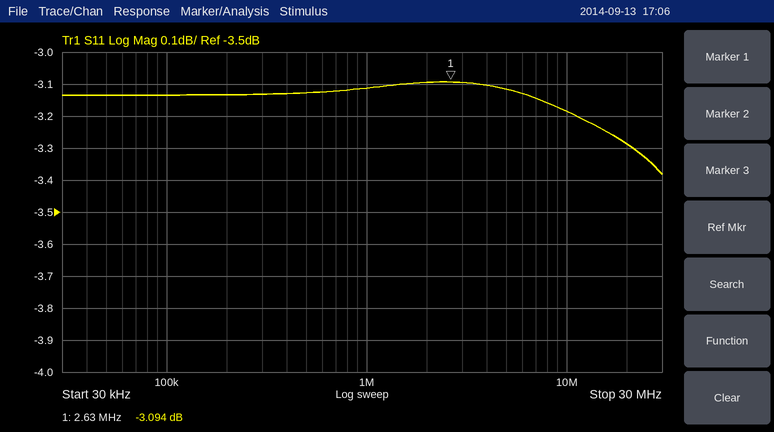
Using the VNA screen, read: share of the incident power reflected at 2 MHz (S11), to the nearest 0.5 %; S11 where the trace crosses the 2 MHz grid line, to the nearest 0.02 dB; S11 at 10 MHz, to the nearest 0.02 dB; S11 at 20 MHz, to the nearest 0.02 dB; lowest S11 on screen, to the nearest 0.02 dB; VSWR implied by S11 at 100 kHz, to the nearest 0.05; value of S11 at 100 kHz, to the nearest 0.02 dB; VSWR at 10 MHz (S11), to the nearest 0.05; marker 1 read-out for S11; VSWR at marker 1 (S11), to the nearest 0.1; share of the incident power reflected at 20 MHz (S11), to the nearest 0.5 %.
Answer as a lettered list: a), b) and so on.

a) 49.0 %
b) -3.10 dB
c) -3.18 dB
d) -3.28 dB
e) -3.38 dB
f) 5.60
g) -3.14 dB
h) 5.50
i) -3.094 dB
j) 5.7
k) 47.0 %
